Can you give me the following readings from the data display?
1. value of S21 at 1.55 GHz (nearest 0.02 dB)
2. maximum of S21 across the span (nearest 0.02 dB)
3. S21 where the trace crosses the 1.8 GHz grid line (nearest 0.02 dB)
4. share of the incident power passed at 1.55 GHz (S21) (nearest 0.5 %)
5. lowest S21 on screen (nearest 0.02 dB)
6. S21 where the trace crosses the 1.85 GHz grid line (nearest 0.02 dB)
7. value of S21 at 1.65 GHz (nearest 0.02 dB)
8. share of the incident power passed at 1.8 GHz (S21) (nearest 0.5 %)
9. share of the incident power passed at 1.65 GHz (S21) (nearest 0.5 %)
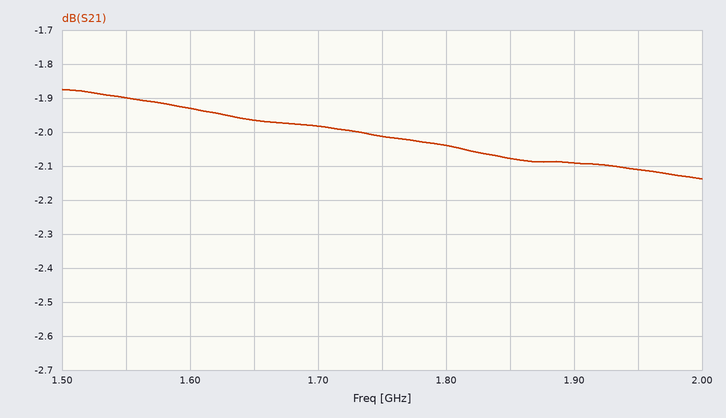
-1.90 dB
-1.88 dB
-2.04 dB
64.5 %
-2.14 dB
-2.08 dB
-1.96 dB
62.5 %
63.5 %
